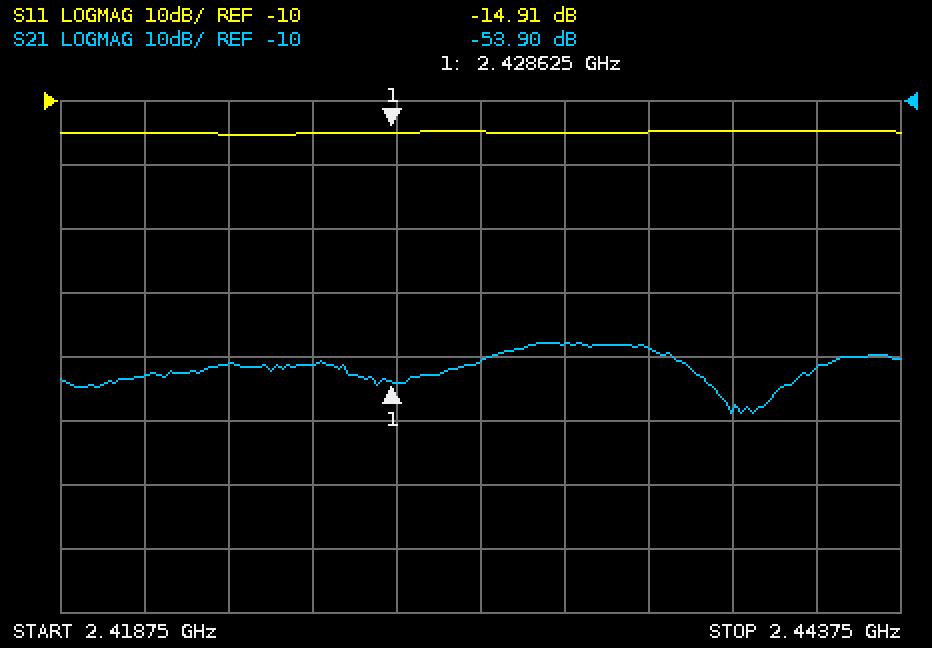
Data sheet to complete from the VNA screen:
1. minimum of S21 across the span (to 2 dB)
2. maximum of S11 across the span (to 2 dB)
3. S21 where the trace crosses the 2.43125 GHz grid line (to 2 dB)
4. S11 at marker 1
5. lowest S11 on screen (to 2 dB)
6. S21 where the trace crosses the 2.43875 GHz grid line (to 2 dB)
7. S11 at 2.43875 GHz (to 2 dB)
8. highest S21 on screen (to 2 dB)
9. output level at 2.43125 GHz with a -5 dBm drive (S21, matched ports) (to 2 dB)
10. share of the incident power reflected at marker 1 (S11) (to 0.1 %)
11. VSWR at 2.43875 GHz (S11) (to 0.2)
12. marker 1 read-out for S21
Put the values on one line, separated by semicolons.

-58 dB; -14 dB; -50 dB; -14.91 dB; -16 dB; -58 dB; -14 dB; -48 dB; -56 dBm; 3.2 %; 1.4; -53.90 dB
